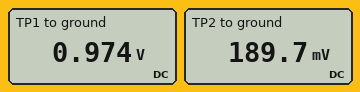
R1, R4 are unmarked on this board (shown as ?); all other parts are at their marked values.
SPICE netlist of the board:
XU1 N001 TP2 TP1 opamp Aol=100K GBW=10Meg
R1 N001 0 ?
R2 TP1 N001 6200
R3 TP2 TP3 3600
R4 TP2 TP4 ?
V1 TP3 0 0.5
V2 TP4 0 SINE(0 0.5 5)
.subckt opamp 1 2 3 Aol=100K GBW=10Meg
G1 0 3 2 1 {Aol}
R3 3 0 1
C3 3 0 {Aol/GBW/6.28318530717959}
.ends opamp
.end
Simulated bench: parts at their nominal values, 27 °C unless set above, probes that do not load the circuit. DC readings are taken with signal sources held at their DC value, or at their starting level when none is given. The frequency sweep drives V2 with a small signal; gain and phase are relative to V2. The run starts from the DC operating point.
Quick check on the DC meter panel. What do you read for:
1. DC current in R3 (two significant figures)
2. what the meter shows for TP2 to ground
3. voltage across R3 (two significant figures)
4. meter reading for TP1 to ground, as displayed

86 µA
189.7 mV
310 mV
0.974 V
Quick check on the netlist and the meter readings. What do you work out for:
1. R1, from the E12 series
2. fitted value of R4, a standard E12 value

1.5 kΩ
2.2 kΩ
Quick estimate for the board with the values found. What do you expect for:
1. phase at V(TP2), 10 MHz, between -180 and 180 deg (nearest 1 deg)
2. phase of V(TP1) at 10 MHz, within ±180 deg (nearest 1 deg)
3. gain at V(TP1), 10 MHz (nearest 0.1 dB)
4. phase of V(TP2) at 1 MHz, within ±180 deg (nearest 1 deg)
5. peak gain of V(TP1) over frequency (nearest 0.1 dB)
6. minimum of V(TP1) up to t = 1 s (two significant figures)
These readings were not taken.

0 deg
-79 deg
-4.3 dB
0 deg
10.1 dB
-620 mV
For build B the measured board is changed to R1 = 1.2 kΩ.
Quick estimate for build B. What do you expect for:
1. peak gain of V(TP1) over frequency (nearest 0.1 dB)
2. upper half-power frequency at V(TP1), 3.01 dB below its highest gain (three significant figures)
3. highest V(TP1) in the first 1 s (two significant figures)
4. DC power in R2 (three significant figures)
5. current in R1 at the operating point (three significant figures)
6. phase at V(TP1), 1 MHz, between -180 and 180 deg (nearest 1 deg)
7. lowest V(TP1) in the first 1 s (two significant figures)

11.7 dB
1.62 MHz
3.1 V
155 µW
158 µA
-32 deg
-740 mV
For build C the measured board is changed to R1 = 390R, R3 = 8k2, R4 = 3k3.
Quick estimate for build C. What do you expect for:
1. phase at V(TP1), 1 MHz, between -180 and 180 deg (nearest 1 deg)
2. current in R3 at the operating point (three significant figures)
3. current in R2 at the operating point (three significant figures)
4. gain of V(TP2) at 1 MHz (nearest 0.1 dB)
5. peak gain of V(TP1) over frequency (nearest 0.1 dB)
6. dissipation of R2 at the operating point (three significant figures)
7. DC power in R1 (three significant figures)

-59 deg
43.5 µA
368 µA
-2.9 dB
21.6 dB
839 µW
52.8 µW
